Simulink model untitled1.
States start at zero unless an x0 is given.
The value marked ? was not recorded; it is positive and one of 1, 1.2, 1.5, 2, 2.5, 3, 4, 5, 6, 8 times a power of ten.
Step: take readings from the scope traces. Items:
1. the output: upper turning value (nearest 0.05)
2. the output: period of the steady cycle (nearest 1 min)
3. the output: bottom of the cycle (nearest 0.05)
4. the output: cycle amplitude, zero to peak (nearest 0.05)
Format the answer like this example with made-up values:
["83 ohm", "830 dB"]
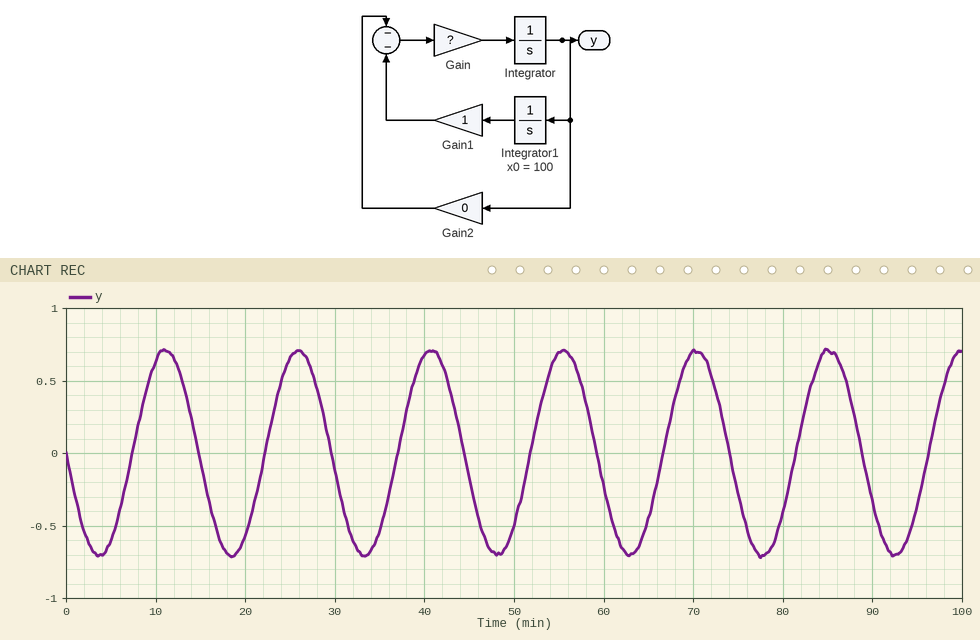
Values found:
["0.70", "15 min", "-0.70", "0.70"]
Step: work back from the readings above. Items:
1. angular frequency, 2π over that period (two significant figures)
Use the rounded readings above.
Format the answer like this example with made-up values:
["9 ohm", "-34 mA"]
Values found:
["0.42 rad/min"]
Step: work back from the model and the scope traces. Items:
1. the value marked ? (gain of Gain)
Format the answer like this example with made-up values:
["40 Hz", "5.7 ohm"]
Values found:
["5e-05"]
